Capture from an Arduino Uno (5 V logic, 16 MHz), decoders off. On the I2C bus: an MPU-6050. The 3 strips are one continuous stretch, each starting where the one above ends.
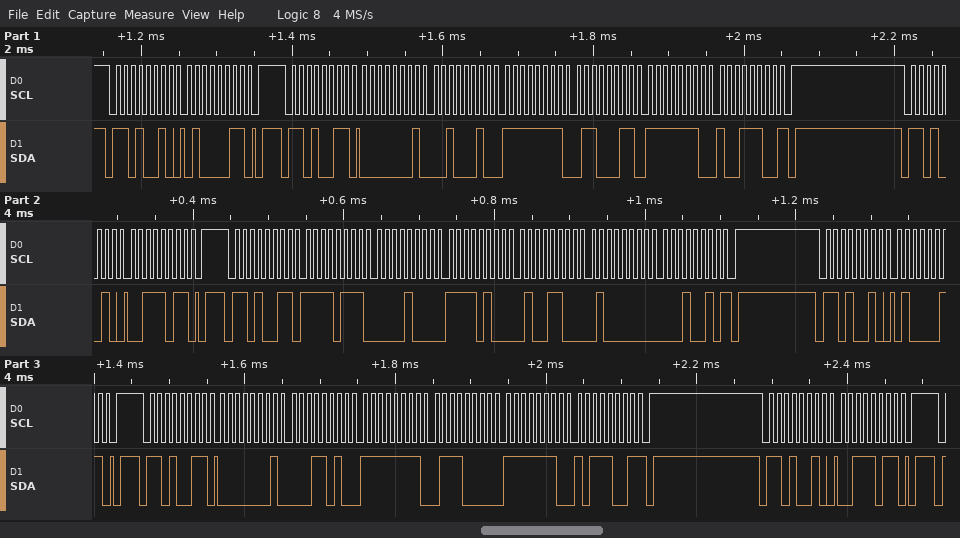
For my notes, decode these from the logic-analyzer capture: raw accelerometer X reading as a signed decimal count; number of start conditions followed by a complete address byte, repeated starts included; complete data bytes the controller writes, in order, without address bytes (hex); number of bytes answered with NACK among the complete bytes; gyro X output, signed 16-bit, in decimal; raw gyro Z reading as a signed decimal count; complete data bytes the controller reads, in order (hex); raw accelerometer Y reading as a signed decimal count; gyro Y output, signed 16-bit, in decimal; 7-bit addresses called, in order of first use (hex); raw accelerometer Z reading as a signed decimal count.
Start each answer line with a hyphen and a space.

- -2296
- 7
- 43 3B 43 3B
- 3
- 290
- -356
- 01 22 FF 63 FE 9C F7 08 F4 4C 40 12 01 1A FF 70 FE B9
- -2996
- -157
- 0x69
- 16402
